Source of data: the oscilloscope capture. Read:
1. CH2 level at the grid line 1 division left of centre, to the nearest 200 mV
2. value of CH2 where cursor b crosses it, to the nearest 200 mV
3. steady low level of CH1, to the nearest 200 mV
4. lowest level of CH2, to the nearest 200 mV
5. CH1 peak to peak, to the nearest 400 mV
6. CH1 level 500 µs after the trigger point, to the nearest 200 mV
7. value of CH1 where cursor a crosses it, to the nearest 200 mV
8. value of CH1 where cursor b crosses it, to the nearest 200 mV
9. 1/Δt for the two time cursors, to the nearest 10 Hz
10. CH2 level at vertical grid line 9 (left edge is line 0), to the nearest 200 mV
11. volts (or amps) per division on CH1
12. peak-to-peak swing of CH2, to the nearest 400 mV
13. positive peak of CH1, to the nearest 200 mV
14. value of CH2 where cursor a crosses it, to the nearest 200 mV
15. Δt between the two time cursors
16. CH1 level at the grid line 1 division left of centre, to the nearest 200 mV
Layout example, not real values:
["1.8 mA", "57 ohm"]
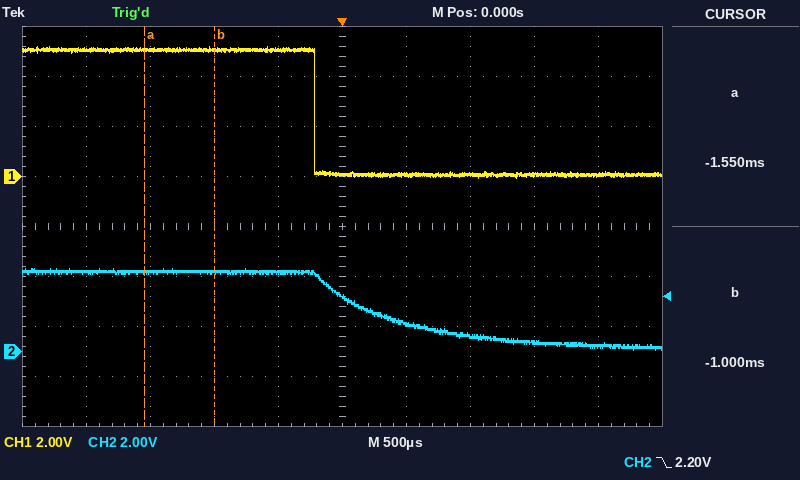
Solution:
["3.2 V", "3.2 V", "0.0 V", "0.0 V", "5.2 V", "0.0 V", "5.0 V", "5.0 V", "1.82 kHz", "200 mV", "2 V", "3.2 V", "5.2 V", "3.2 V", "550 µs", "5.0 V"]
